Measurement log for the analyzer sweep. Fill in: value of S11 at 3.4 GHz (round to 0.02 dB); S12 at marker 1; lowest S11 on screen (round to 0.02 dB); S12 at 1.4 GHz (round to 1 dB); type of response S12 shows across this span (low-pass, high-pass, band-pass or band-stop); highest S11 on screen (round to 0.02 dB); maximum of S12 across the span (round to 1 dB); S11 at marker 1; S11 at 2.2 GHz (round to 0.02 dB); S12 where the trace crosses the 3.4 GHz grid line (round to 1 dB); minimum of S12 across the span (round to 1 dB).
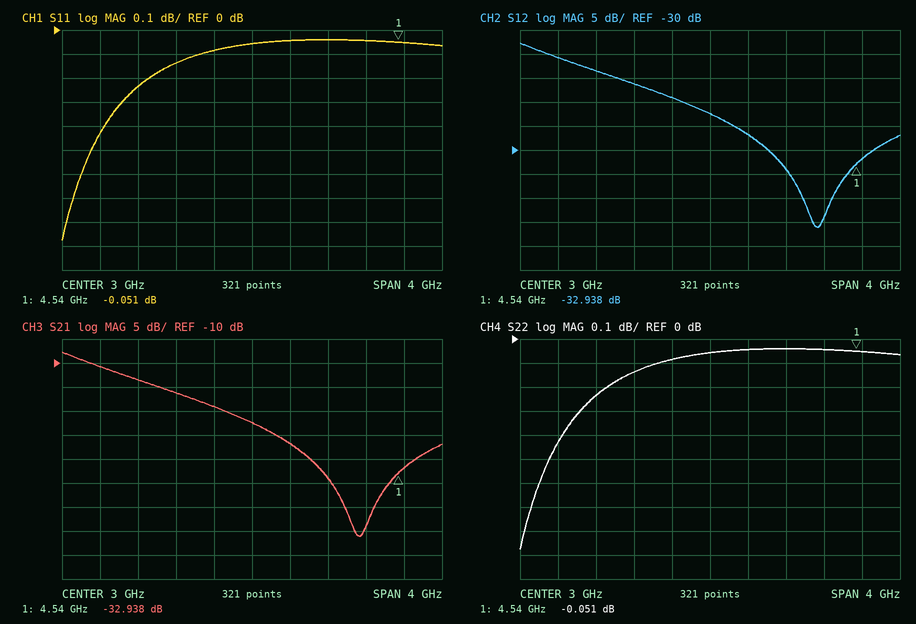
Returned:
-0.04 dB
-32.938 dB
-0.88 dB
-11 dB
low-pass
-0.04 dB
-8 dB
-0.051 dB
-0.14 dB
-27 dB
-46 dB
